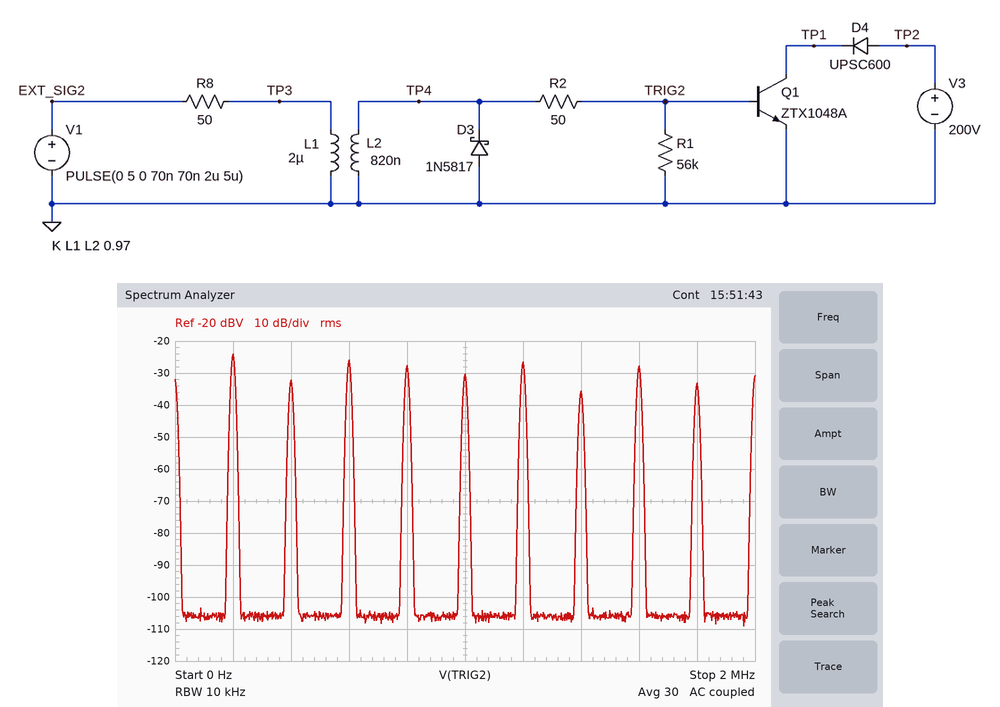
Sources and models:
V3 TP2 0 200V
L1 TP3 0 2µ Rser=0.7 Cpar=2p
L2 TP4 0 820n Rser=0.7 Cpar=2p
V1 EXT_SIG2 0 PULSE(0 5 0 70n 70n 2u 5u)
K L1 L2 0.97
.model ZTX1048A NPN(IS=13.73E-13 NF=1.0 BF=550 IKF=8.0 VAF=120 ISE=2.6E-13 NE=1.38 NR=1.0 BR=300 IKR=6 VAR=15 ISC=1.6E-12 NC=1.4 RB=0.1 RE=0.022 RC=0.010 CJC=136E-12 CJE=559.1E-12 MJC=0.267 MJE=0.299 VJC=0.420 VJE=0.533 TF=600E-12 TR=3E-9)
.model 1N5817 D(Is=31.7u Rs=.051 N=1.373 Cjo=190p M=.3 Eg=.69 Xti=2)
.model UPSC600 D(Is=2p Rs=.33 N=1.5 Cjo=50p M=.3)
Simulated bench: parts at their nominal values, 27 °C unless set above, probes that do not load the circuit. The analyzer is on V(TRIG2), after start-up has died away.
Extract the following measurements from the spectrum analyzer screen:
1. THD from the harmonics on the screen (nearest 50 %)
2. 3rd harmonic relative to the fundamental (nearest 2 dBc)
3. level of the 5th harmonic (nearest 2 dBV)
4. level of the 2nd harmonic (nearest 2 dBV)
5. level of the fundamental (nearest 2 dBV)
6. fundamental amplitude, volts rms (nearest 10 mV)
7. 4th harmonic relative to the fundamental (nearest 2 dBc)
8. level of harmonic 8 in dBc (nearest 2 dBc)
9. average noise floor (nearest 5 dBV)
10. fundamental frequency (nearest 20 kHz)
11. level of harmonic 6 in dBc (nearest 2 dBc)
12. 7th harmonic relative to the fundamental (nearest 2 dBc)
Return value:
150 %
-2 dBc
-30 dBV
-32 dBV
-24 dBV
60 mV
-4 dBc
-4 dBc
-105 dBV
200 kHz
-2 dBc
-12 dBc
